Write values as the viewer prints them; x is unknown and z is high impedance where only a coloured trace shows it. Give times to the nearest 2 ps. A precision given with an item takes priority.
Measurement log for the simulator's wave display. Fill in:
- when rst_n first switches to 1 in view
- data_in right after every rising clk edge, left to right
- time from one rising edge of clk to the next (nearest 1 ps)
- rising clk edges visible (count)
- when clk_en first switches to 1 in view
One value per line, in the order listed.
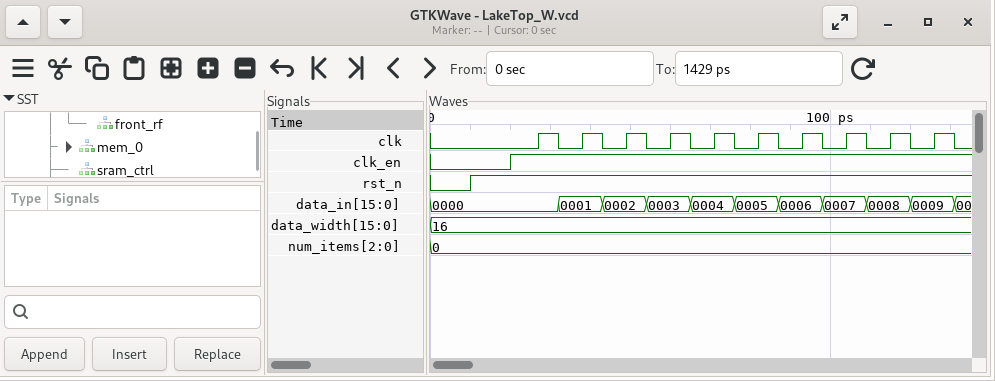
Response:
10 ps
0000, 0001, 0002, 0003, 0004, 0005, 0006, 0007, 0008, 0009
11 ps
10
20 ps
